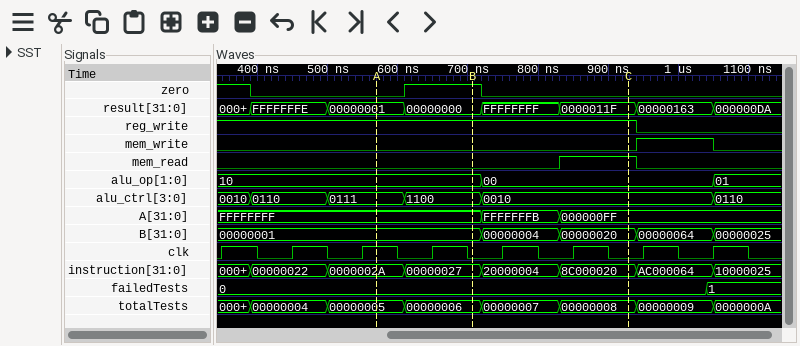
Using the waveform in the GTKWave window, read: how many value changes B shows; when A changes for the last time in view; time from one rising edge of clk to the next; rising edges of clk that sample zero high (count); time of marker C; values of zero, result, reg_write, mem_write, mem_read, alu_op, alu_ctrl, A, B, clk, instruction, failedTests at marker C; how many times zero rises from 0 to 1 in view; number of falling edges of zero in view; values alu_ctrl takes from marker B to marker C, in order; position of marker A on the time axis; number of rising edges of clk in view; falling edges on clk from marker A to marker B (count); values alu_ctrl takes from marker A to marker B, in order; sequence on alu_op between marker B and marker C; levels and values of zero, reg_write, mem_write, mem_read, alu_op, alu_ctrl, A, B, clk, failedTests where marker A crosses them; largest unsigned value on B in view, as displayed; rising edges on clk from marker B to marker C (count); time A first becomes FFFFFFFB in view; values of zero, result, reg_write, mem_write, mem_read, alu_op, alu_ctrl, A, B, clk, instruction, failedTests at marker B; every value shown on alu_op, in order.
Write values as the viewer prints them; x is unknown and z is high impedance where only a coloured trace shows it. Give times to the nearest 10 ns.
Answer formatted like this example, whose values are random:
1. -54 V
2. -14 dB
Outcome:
1. 4
2. 830 ns
3. 100 ns
4. 2
5. 930 ns
6. zero=0, result=0000011F, reg_write=1, mem_write=0, mem_read=1, alu_op=00, alu_ctrl=0010, A=000000FF, B=00000020, clk=0, instruction=8C000020, failedTests=0
7. 1
8. 2
9. 1100, 0010
10. 570 ns
11. 8
12. 2
13. 0111, 1100
14. 10, 00
15. zero=0, reg_write=1, mem_write=0, mem_read=0, alu_op=10, alu_ctrl=0111, A=FFFFFFFF, B=00000001, clk=1, failedTests=0
16. 00000064
17. 2
18. 720 ns
19. zero=1, result=00000000, reg_write=1, mem_write=0, mem_read=0, alu_op=10, alu_ctrl=1100, A=FFFFFFFF, B=00000001, clk=0, instruction=00000027, failedTests=0
20. 10, 00, 01
